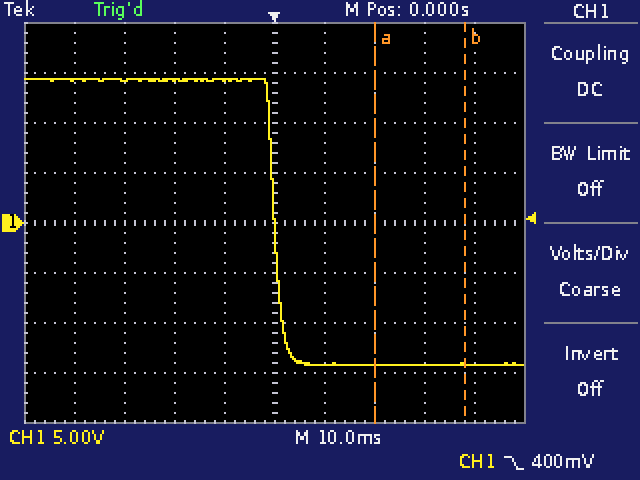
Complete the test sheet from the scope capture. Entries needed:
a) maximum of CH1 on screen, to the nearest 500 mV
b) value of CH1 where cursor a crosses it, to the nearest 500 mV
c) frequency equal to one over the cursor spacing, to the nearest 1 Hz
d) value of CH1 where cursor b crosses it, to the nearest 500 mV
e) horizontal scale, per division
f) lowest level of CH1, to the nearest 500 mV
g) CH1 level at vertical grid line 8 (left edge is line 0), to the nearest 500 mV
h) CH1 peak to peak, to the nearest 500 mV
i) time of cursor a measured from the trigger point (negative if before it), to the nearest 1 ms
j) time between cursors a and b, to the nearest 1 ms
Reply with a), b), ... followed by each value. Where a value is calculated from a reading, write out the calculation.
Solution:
a) 14.5 V
b) -14.0 V
c) 1 / 18 ms ≈ 56 Hz
d) -14.0 V
e) 10 ms
f) -14.0 V
g) -14.0 V
h) 14.5 V − (-14.0 V) = 28.5 V
i) +20 ms
j) 18 ms
